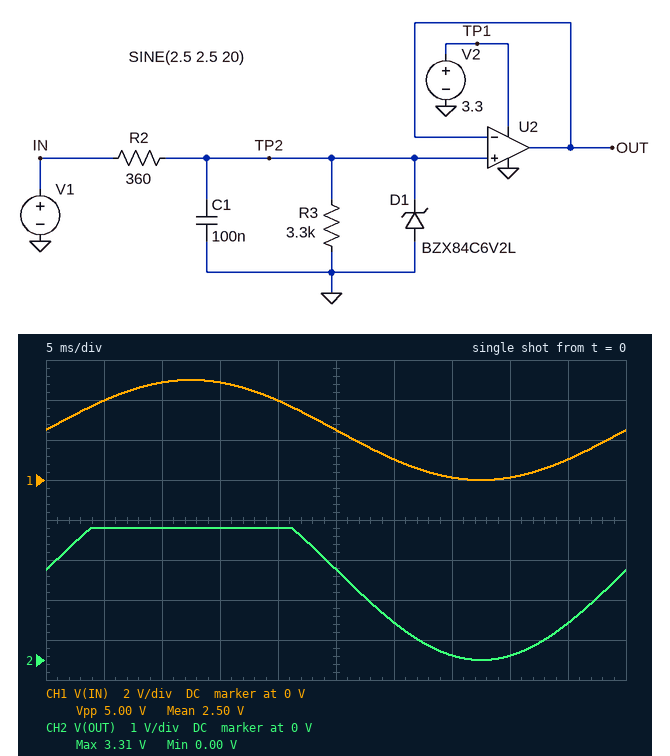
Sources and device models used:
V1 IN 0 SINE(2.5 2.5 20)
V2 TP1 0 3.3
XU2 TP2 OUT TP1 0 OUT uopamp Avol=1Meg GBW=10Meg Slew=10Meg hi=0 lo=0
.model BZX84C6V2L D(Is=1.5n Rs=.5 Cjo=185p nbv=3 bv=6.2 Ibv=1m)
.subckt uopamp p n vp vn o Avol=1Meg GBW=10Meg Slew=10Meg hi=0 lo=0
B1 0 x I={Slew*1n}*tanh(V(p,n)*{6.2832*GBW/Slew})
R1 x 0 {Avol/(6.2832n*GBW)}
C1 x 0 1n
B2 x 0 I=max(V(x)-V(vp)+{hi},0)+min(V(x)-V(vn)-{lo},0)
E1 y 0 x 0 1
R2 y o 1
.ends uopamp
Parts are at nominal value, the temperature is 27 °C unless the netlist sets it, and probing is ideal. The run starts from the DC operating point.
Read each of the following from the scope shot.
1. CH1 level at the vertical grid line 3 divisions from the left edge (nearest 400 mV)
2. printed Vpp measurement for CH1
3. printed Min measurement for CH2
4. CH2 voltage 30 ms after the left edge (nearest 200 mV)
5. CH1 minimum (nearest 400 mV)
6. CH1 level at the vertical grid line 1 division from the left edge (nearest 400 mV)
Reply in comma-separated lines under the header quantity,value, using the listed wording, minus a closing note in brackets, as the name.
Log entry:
quantity,value
CH1 level at the vertical grid line 3 divisions from the left edge,4.8 V
printed Vpp measurement for CH1,5.00 V
printed Min measurement for CH2,0.00 V
CH2 voltage 30 ms after the left edge,1.0 V
CH1 minimum,0 V
CH1 level at the vertical grid line 1 division from the left edge,4.0 V
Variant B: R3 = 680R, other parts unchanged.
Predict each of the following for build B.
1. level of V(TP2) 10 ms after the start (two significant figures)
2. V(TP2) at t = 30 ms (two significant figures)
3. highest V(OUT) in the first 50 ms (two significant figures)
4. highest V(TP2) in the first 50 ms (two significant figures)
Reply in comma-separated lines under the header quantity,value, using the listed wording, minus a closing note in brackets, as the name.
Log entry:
quantity,value
level of V(TP2) 10 ms after the start,3.2 V
V(TP2) at t = 30 ms,680 mV
highest V(OUT) in the first 50 ms,3.3 V
highest V(TP2) in the first 50 ms,3.3 V
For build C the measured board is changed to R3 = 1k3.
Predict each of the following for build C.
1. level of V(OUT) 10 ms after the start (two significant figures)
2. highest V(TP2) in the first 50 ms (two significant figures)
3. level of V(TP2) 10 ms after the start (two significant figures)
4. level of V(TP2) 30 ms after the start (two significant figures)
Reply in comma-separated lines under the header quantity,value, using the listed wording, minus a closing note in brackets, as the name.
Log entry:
quantity,value
level of V(OUT) 10 ms after the start,3.3 V
highest V(TP2) in the first 50 ms,3.9 V
level of V(TP2) 10 ms after the start,3.8 V
level of V(TP2) 30 ms after the start,810 mV
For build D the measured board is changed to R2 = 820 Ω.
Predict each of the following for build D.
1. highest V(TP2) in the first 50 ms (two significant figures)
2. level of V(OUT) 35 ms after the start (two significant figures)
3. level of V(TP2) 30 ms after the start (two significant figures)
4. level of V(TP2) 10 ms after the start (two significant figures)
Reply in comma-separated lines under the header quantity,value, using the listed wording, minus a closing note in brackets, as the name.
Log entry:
quantity,value
highest V(TP2) in the first 50 ms,4.0 V
level of V(OUT) 35 ms after the start,100 mV
level of V(TP2) 30 ms after the start,840 mV
level of V(TP2) 10 ms after the start,3.9 V
